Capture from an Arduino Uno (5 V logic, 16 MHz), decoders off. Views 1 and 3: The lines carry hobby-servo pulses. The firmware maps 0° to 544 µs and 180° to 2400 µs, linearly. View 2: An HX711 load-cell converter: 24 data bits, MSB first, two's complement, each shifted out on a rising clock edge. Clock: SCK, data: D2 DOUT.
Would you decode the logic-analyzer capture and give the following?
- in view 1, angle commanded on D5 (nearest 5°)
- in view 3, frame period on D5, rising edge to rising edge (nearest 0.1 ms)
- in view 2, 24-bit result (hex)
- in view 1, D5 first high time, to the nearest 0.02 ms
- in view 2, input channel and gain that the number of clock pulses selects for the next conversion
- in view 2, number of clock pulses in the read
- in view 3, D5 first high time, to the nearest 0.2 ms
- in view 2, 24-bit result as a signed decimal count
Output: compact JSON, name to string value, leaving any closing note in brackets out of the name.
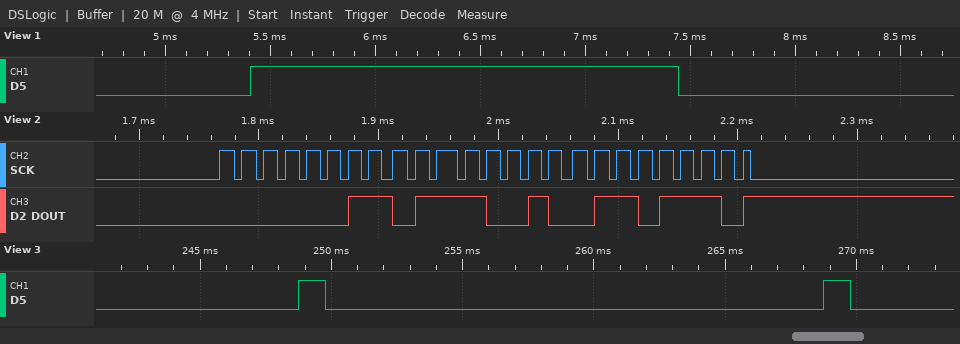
{"in view 1, angle commanded on D5": "145°", "in view 3, frame period on D5, rising edge to rising edge": "20.0 ms", "in view 2, 24-bit result": "0x03726E", "in view 1, D5 first high time, to the nearest 0.02 ms": "2.04 ms", "in view 2, input channel and gain that the number of clock pulses selects for the next conversion": "channel A, gain 128", "in view 2, number of clock pulses in the read": "25", "in view 3, D5 first high time, to the nearest 0.2 ms": "1.0 ms", "in view 2, 24-bit result as a signed decimal count": "225902"}
